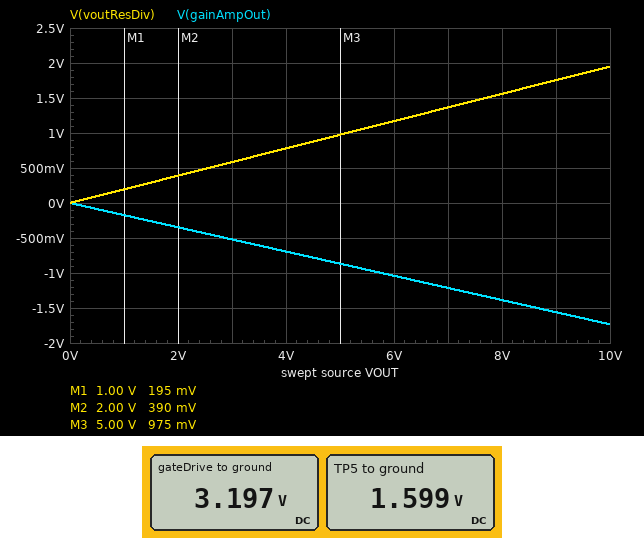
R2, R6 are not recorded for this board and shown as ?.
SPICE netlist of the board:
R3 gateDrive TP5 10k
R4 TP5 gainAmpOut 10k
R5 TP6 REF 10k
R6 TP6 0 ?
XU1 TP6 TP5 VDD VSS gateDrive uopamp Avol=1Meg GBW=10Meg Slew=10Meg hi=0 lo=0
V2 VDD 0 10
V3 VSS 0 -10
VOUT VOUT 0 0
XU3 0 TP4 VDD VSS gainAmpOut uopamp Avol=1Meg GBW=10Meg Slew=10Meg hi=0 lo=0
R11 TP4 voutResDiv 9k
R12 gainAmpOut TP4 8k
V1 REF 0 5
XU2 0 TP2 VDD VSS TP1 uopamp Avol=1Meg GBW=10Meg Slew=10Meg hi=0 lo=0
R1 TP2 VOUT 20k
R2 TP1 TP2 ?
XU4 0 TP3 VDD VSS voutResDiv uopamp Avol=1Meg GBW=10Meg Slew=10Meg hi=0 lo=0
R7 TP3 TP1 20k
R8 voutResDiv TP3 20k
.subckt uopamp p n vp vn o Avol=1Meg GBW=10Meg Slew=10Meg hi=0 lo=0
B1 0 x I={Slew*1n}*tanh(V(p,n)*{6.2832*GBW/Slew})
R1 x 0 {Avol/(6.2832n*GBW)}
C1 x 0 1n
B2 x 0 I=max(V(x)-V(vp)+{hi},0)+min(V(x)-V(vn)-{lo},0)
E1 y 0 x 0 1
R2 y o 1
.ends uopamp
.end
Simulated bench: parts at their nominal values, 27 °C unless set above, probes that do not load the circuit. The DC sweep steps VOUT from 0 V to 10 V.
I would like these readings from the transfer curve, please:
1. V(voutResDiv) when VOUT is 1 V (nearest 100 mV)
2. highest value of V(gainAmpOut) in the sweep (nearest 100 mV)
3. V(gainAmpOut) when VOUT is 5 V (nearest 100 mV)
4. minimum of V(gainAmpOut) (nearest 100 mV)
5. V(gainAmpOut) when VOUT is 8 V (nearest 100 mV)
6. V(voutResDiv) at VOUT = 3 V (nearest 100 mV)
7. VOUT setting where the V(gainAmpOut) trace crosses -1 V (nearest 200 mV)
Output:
200 mV
0 V
-900 mV
-1.7 V
-1.4 V
600 mV
5.8 V
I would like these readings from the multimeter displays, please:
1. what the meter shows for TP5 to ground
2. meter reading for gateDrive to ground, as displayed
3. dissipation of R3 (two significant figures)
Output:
1.599 V
3.197 V
260 µW
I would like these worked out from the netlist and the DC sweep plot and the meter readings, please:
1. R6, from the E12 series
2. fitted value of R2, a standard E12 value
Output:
4.7 kΩ
3.9 kΩ
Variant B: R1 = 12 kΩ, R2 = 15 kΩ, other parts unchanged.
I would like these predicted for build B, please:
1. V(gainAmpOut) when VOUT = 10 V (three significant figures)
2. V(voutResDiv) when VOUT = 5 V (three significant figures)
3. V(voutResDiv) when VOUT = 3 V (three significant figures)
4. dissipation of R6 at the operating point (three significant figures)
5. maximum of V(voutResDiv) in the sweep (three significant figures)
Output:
-8.89 V
6.25 V
3.75 V
544 µW
10.0 V
